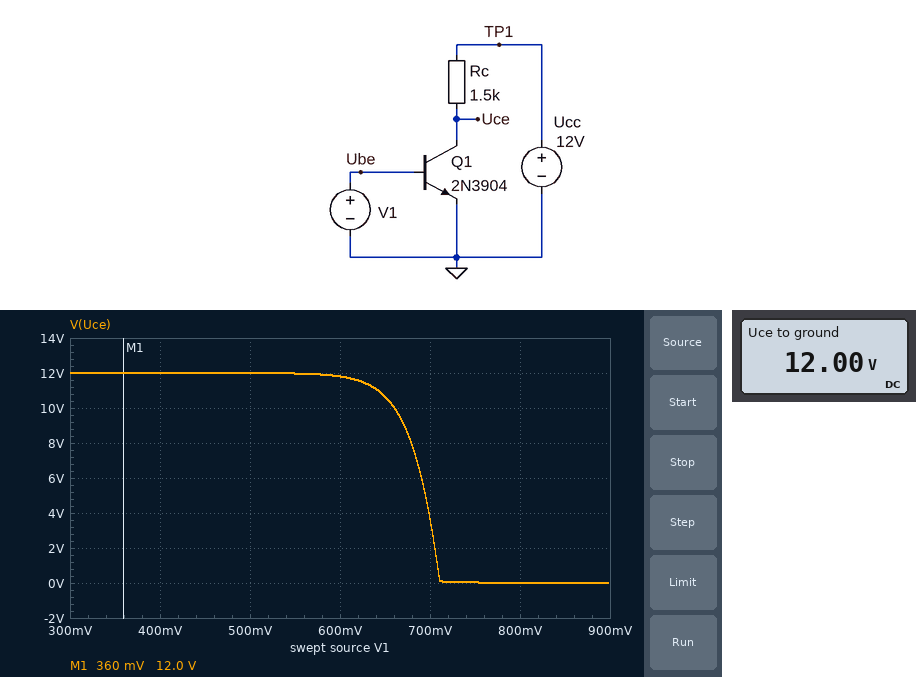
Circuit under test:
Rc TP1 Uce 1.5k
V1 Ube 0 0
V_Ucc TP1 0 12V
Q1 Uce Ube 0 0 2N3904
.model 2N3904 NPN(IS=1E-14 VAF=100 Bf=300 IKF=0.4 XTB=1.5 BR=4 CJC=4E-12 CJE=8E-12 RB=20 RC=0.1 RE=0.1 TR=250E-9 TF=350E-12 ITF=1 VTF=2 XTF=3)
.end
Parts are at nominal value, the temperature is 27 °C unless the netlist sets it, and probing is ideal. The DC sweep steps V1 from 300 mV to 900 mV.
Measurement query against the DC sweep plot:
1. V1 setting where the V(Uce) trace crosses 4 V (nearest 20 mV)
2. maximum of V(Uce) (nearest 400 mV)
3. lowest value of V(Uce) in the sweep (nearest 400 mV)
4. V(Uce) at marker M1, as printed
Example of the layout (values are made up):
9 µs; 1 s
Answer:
700 mV; 12.0 V; 0 V; 12.0 V
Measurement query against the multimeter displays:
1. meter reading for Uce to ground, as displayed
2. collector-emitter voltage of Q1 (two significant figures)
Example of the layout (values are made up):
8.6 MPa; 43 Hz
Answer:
12.00 V; 12 V
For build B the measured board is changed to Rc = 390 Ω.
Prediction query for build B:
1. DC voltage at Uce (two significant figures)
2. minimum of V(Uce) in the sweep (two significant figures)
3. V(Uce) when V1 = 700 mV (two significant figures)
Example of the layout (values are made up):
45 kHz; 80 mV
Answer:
12 V; 32 mV; 9.7 V
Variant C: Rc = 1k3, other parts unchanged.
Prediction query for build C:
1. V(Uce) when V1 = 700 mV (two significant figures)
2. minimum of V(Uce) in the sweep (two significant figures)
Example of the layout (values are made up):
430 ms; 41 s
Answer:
4.7 V; 15 mV
